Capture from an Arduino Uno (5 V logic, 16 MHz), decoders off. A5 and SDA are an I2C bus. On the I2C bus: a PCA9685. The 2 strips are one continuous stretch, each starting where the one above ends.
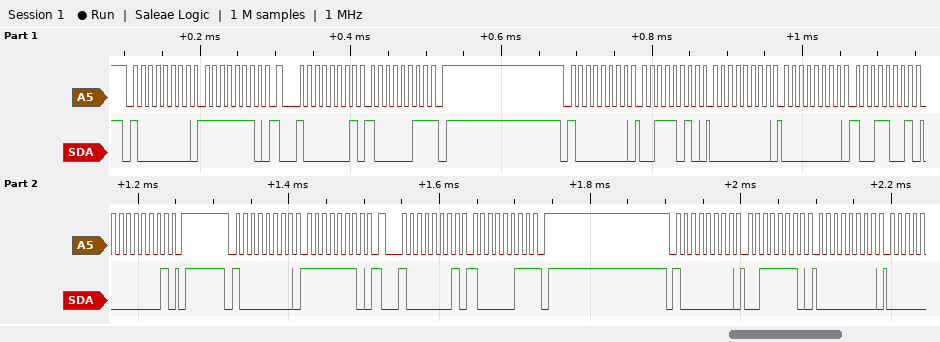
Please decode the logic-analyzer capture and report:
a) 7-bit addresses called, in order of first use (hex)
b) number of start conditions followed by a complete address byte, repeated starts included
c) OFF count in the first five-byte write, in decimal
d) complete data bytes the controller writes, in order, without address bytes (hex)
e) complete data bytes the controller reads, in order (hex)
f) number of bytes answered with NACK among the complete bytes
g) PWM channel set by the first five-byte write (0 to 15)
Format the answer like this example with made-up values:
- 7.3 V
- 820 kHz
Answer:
- 0x40
- 6
- 409
- FE 3A 00 00 99 01 FE 3E 00
- 83 83
- 2
- 13
